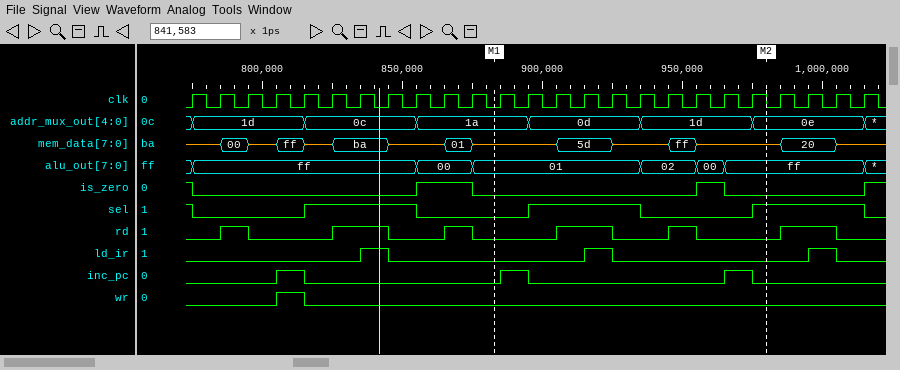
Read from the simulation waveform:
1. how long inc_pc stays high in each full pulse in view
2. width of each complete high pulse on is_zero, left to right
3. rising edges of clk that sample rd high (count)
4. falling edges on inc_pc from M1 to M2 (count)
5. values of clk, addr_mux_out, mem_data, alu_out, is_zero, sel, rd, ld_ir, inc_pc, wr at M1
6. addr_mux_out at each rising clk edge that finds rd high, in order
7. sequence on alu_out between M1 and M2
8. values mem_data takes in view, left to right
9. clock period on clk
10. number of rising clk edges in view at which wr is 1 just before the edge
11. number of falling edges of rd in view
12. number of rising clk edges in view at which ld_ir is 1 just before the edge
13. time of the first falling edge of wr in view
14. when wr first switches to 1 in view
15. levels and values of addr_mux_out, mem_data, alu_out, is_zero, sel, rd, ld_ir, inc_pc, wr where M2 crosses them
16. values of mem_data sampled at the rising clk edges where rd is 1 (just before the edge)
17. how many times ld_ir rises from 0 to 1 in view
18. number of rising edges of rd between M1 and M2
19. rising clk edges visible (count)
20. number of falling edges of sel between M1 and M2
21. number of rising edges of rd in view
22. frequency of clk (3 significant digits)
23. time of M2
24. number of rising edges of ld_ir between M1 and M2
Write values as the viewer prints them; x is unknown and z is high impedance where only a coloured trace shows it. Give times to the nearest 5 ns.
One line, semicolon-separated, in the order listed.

10 ns, 10 ns, 10 ns; 20 ns, 10 ns; 9; 2; clk=0, addr_mux_out=1a, mem_data=z, alu_out=01, is_zero=0, sel=0, rd=0, ld_ir=0, inc_pc=0, wr=0; 1d, 0c, 0c, 1a, 0d, 0d, 1d, 0e, 0e; 01, 02, 00, ff; z, 00, z, ff, z, ba, z, 01, z, 5d, z, ff, z, 20, z; 10 ns; 1; 6; 3; 815 ns; 805 ns; addr_mux_out=0e, mem_data=z, alu_out=ff, is_zero=0, sel=1, rd=0, ld_ir=0, inc_pc=0, wr=0; 00, ba, ba, 01, 5d, 5d, ff, 20, 20; 3; 2; 25; 1; 6; 100 MHz; 980 ns; 1
